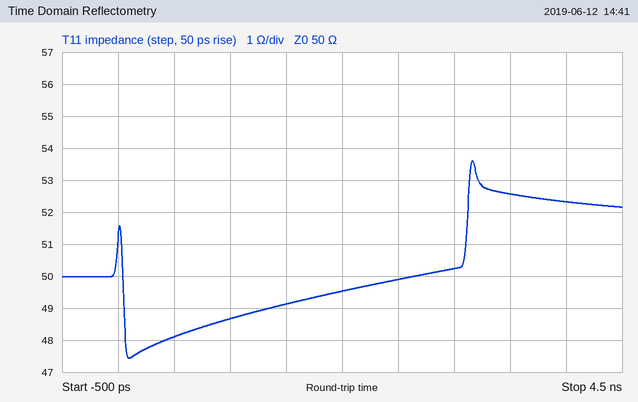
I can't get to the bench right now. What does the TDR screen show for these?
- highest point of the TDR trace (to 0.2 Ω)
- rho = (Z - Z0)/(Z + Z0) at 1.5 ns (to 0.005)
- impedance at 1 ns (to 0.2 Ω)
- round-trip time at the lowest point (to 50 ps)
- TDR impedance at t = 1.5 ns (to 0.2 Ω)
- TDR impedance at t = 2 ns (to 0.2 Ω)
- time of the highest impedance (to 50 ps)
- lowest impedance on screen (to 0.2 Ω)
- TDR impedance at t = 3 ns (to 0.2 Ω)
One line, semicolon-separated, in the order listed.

53.6 Ω; -0.010; 48.6 Ω; 100 ps; 49.2 Ω; 49.6 Ω; 3.15 ns; 47.4 Ω; 50.2 Ω
